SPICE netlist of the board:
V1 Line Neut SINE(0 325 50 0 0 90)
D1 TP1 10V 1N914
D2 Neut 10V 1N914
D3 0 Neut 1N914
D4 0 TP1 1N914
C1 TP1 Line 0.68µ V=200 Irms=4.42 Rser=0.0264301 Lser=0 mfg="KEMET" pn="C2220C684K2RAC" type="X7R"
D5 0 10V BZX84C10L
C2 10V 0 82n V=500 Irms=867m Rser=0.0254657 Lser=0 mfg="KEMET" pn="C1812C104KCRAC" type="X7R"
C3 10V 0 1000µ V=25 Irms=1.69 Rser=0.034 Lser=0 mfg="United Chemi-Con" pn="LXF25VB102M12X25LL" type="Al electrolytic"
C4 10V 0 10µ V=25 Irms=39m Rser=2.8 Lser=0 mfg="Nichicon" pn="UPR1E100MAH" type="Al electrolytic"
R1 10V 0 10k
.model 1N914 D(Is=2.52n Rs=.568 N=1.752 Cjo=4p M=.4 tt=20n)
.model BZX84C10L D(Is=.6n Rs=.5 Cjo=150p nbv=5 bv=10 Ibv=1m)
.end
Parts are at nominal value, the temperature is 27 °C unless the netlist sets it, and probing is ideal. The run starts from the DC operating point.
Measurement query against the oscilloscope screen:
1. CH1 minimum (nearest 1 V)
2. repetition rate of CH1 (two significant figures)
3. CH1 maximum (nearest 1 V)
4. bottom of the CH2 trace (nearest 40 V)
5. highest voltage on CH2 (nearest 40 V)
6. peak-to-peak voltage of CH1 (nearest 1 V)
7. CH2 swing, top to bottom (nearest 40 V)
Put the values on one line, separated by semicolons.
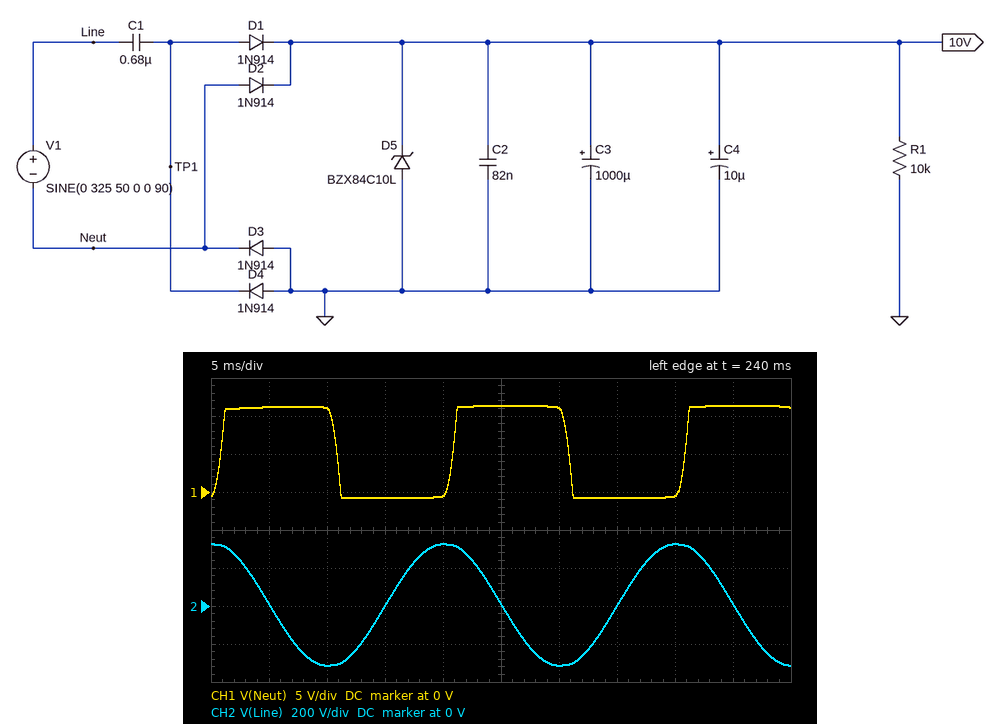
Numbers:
-1 V; 50 Hz; 11 V; -320 V; 320 V; 12 V; 640 V
